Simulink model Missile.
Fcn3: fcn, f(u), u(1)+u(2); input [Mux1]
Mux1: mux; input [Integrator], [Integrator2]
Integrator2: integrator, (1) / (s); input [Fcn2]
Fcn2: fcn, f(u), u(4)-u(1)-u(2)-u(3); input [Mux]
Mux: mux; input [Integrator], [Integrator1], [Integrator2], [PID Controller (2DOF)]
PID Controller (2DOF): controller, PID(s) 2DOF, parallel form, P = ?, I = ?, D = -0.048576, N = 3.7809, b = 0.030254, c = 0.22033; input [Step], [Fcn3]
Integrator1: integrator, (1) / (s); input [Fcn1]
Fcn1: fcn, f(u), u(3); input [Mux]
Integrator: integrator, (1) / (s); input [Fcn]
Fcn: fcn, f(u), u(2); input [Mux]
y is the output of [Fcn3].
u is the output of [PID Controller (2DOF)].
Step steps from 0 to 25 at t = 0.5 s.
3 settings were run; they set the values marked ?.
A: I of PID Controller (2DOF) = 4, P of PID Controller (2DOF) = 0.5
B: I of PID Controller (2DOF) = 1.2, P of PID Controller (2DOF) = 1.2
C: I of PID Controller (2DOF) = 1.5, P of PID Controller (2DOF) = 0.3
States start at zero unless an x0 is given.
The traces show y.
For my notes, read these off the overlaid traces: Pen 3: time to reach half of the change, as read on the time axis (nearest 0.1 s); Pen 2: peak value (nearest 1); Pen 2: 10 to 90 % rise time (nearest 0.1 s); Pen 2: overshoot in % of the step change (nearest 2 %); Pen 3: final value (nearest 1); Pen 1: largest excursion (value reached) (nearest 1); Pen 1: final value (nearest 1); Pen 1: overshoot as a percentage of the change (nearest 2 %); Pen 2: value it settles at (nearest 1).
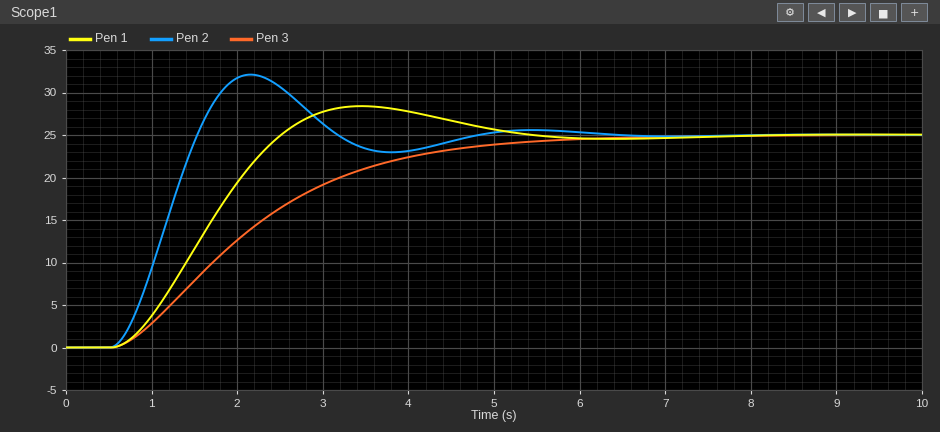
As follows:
2.0 s
32
0.7 s
28 %
25
28
25
14 %
25
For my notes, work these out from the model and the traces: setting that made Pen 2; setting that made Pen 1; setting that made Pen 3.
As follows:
A
C
B
